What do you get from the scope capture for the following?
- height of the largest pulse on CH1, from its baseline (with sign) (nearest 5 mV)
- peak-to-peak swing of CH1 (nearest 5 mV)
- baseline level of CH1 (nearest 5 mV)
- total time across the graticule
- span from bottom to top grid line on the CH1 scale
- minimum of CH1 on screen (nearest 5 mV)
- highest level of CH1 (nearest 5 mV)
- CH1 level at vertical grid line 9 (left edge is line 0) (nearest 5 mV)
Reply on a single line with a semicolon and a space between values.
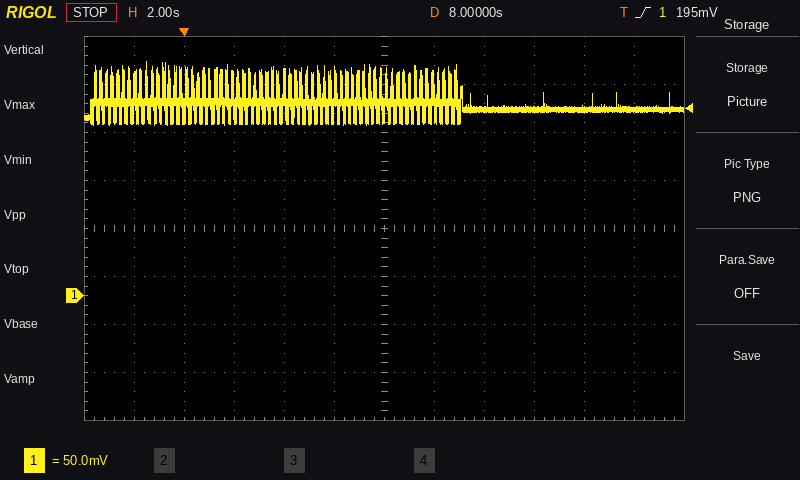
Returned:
+50 mV; 65 mV; 195 mV; 24 s; 400 mV; 180 mV; 245 mV; 195 mV
